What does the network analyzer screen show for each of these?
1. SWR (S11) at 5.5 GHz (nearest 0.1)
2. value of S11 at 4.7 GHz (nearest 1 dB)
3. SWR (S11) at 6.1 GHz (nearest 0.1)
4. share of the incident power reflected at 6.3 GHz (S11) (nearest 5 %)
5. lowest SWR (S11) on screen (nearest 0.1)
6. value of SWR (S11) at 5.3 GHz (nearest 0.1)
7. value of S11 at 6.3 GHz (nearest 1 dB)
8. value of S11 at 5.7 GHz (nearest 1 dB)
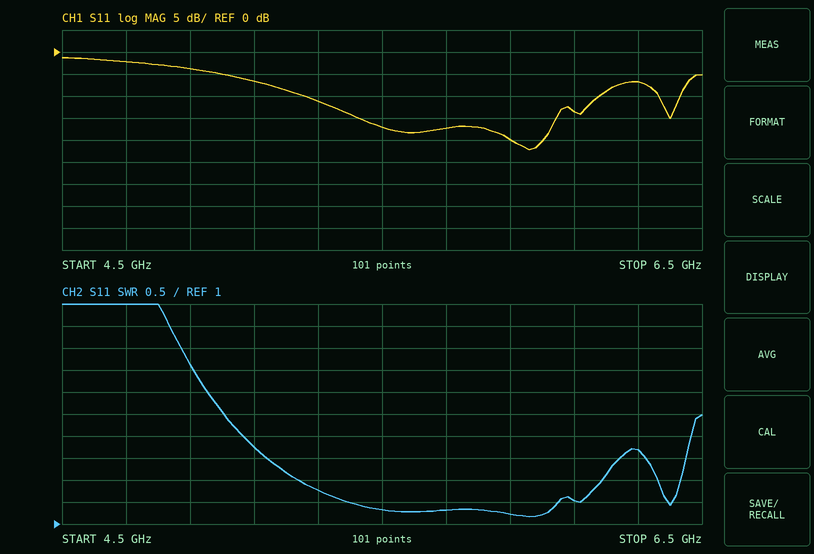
1.3
-2 dB
1.5
20 %
1.2
1.8
-7 dB
-17 dB
